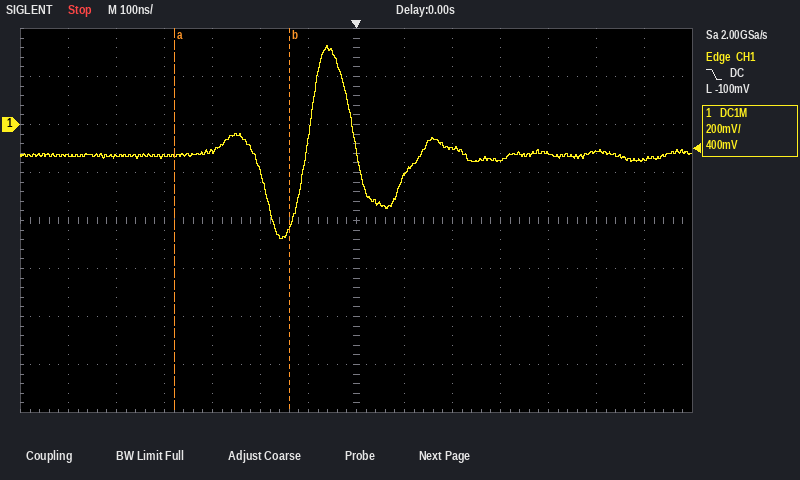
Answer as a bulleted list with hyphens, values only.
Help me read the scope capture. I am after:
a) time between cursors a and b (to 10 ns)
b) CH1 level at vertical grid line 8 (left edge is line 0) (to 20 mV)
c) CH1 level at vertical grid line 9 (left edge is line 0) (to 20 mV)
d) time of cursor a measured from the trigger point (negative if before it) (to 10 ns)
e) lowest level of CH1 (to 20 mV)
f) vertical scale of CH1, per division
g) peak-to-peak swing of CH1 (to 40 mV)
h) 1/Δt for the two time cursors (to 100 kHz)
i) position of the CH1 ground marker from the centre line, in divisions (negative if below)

- 240 ns
- -220 mV
- -100 mV
- -380 ns
- -480 mV
- 200 mV
- 800 mV
- 4.2 MHz
- +2.0 div
